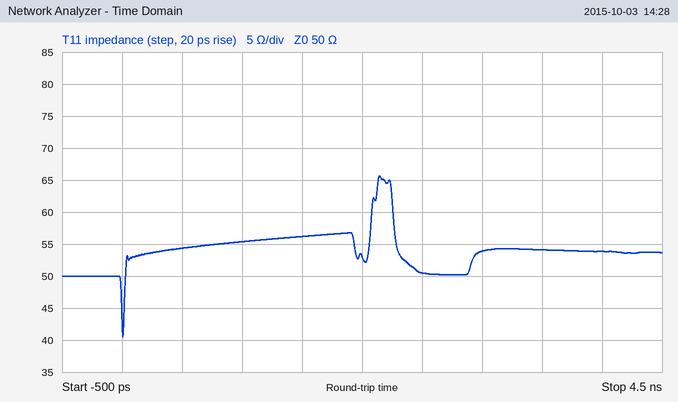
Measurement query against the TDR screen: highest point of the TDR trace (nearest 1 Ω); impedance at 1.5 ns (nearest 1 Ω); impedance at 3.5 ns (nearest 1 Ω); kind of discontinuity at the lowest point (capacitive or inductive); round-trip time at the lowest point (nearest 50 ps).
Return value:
66 Ω
56 Ω
54 Ω
capacitive
0 ps
